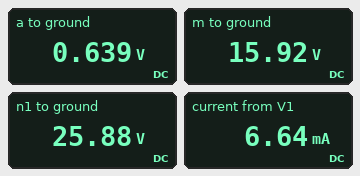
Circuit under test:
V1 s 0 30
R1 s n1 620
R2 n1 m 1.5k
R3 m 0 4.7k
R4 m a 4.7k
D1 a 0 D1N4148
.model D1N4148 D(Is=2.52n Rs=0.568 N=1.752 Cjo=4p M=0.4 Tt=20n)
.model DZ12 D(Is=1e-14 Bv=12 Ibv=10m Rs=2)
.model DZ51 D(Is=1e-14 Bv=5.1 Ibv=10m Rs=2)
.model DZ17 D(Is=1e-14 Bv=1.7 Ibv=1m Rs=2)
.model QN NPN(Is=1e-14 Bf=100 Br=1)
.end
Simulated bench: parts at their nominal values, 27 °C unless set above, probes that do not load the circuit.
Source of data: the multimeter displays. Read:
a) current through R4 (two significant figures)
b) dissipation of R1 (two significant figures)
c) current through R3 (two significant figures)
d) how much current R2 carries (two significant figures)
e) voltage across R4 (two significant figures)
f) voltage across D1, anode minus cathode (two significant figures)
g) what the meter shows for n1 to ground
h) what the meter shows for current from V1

3.3 mA
27 mW
3.4 mA
6.6 mA
15 V
640 mV
25.88 V
6.64 mA
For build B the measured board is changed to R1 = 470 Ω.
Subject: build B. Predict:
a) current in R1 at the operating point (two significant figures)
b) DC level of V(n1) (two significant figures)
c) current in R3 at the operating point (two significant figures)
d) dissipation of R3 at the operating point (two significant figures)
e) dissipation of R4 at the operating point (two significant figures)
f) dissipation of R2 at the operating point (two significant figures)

6.9 mA
27 V
3.5 mA
58 mW
53 mW
71 mW
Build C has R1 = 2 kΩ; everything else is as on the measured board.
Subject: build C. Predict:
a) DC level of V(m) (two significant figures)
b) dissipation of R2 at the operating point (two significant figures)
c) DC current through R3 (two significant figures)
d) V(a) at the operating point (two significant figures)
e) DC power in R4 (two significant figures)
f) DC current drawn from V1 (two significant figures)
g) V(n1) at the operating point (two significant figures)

12 V
39 mW
2.6 mA
630 mV
29 mW
5.1 mA
20 V
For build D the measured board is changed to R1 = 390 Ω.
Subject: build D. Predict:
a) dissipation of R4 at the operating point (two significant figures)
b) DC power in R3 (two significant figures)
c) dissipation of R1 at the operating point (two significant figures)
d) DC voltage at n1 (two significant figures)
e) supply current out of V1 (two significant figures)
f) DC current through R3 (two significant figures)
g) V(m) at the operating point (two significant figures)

55 mW
60 mW
19 mW
27 V
7.0 mA
3.6 mA
17 V
